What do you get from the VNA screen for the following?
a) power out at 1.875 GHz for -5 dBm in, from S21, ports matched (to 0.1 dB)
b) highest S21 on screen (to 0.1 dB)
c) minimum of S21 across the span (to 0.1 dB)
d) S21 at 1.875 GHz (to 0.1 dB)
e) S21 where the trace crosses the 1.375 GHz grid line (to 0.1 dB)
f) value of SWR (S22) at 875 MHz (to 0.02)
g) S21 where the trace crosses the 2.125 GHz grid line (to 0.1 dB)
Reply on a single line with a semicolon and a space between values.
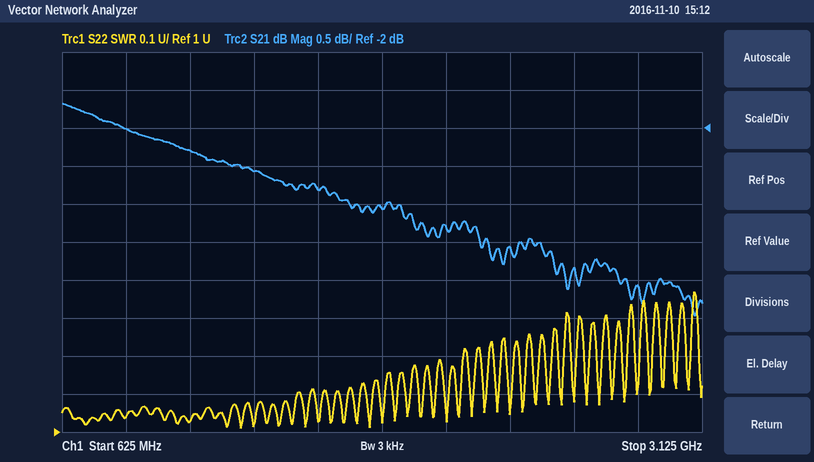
-8.1 dBm; -1.7 dB; -4.5 dB; -3.1 dB; -2.6 dB; 1.04; -3.3 dB
